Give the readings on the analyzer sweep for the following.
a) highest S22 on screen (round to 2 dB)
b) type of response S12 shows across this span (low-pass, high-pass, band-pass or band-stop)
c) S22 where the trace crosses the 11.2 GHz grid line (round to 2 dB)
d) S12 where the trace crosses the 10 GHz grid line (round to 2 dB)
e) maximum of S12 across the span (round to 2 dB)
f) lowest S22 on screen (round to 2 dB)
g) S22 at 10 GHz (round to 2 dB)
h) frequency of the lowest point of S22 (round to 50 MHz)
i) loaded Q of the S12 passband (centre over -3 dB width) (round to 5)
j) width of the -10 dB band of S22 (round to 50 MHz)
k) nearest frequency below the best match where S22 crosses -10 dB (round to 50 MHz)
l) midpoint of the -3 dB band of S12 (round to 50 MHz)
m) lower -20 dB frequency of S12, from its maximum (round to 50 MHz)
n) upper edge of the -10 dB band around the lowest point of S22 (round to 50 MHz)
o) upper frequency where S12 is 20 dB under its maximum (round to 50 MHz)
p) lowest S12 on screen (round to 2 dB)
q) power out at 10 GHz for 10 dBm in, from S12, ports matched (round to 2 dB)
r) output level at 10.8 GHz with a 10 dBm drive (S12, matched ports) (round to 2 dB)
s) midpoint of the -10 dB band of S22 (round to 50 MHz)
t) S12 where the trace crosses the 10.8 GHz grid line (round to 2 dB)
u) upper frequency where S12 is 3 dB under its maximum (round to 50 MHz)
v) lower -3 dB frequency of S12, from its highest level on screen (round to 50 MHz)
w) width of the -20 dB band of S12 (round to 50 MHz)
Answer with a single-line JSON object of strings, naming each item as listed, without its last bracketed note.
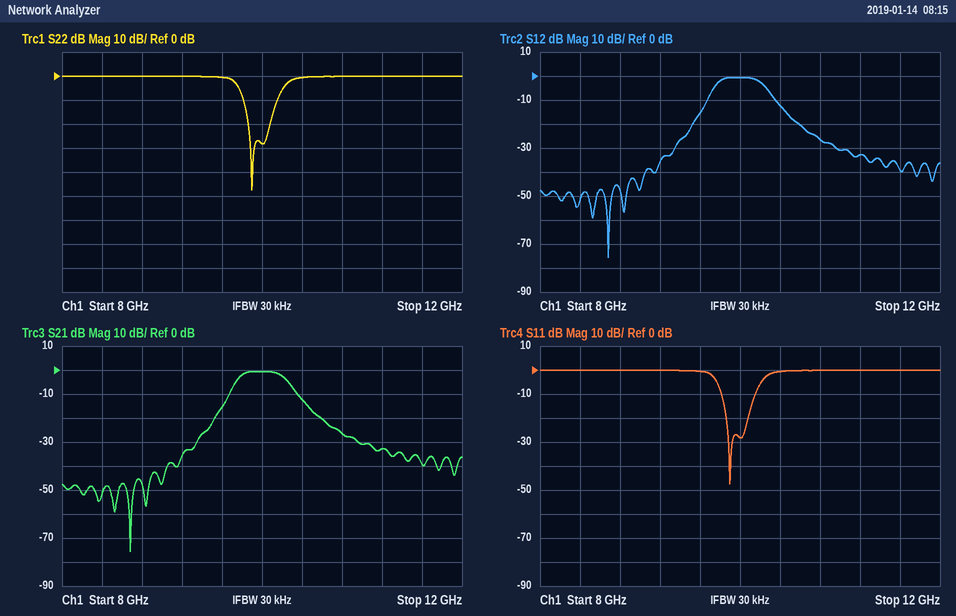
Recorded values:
{"highest S22 on screen": "0 dB", "type of response S12 shows across this span": "band-pass", "S22 where the trace crosses the 11.2 GHz grid line": "0 dB", "S12 where the trace crosses the 10 GHz grid line": "0 dB", "maximum of S12 across the span": "0 dB", "lowest S22 on screen": "-48 dB", "S22 at 10 GHz": "-28 dB", "frequency of the lowest point of S22": "9.90 GHz", "loaded Q of the S12 passband (centre over -3 dB width)": "20", "width of the -10 dB band of S22": "350 MHz", "nearest frequency below the best match where S22 crosses -10 dB": "9.80 GHz", "midpoint of the -3 dB band of S12": "10.00 GHz", "lower -20 dB frequency of S12, from its maximum": "9.50 GHz", "upper edge of the -10 dB band around the lowest point of S22": "10.15 GHz", "upper frequency where S12 is 20 dB under its maximum": "10.60 GHz", "lowest S12 on screen": "-76 dB", "power out at 10 GHz for 10 dBm in, from S12, ports matched": "10 dBm", "output level at 10.8 GHz with a 10 dBm drive (S12, matched ports)": "-16 dBm", "midpoint of the -10 dB band of S22": "10.00 GHz", "S12 where the trace crosses the 10.8 GHz grid line": "-26 dB", "upper frequency where S12 is 3 dB under its maximum": "10.25 GHz", "lower -3 dB frequency of S12, from its highest level on screen": "9.75 GHz", "width of the -20 dB band of S12": "1.10 GHz"}
